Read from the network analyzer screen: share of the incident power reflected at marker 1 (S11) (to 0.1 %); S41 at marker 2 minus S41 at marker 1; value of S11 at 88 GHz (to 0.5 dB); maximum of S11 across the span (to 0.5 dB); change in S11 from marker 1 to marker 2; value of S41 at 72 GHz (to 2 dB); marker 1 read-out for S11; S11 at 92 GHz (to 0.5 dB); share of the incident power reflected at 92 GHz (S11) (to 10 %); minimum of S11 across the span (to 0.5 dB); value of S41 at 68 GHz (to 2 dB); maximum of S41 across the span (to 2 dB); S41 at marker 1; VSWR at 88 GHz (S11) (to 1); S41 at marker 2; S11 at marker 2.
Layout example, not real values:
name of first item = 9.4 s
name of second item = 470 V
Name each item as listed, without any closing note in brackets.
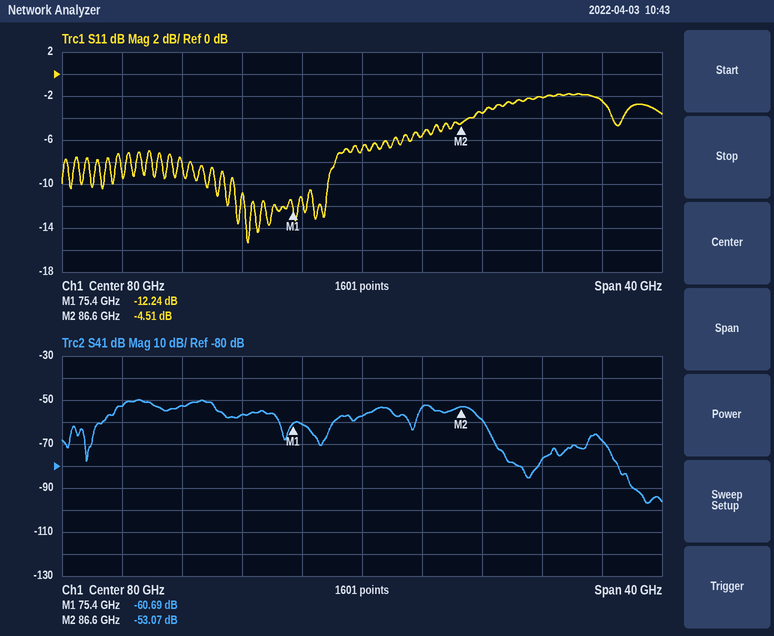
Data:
share of the incident power reflected at marker 1 (S11) = 6.0 %
S41 at marker 2 minus S41 at marker 1 = 7.62 dB
value of S11 at 88 GHz = -3.5 dB
maximum of S11 across the span = -2.0 dB
change in S11 from marker 1 to marker 2 = 7.73 dB
value of S41 at 72 GHz = -56 dB
marker 1 read-out for S11 = -12.24 dB
S11 at 92 GHz = -2.0 dB
share of the incident power reflected at 92 GHz (S11) = 60 %
minimum of S11 across the span = -15.5 dB
value of S41 at 68 GHz = -52 dB
maximum of S41 across the span = -50 dB
S41 at marker 1 = -60.69 dB
VSWR at 88 GHz (S11) = 5
S41 at marker 2 = -53.07 dB
S11 at marker 2 = -4.51 dB
